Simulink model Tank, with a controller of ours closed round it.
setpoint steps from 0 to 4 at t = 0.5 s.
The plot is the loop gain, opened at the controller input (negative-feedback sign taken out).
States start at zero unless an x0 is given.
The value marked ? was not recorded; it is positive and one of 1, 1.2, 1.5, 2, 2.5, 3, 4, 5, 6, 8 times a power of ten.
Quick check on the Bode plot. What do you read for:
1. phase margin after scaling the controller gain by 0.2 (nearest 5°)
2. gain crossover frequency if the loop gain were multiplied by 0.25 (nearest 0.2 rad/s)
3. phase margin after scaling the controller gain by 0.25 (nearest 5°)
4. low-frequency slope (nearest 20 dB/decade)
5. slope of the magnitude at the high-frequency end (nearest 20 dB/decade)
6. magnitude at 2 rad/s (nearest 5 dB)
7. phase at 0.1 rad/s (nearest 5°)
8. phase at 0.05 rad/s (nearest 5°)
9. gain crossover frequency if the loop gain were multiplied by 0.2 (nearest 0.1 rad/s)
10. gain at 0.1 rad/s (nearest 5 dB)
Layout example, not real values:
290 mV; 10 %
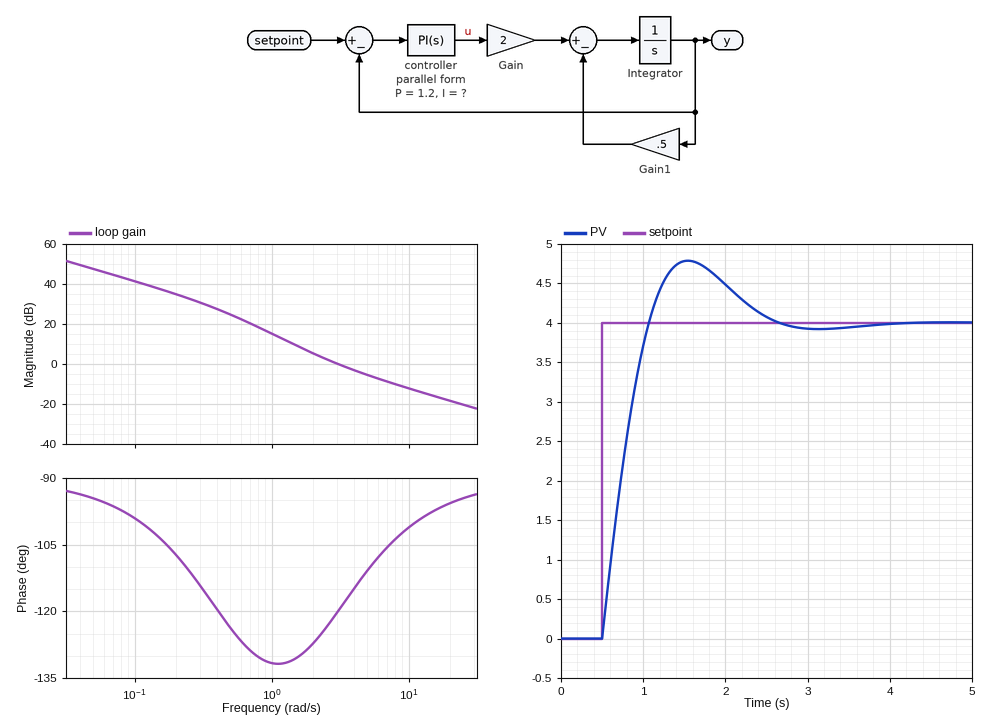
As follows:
50°; 1.2 rad/s; 50°; -20 dB/decade; -20 dB/decade; 5 dB; -100°; -95°; 1.1 rad/s; 40 dB
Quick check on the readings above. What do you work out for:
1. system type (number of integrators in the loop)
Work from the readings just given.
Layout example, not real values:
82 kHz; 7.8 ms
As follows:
1
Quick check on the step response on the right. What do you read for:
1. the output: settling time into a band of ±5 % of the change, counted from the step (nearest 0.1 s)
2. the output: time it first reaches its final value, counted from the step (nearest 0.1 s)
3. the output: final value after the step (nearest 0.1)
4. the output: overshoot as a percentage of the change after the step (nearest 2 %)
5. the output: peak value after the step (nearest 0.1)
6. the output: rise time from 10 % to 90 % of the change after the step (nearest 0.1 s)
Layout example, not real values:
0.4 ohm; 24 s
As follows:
1.8 s; 0.6 s; 4.0; 20 %; 4.8; 0.4 s
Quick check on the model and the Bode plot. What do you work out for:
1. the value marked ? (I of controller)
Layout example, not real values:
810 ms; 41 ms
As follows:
3
